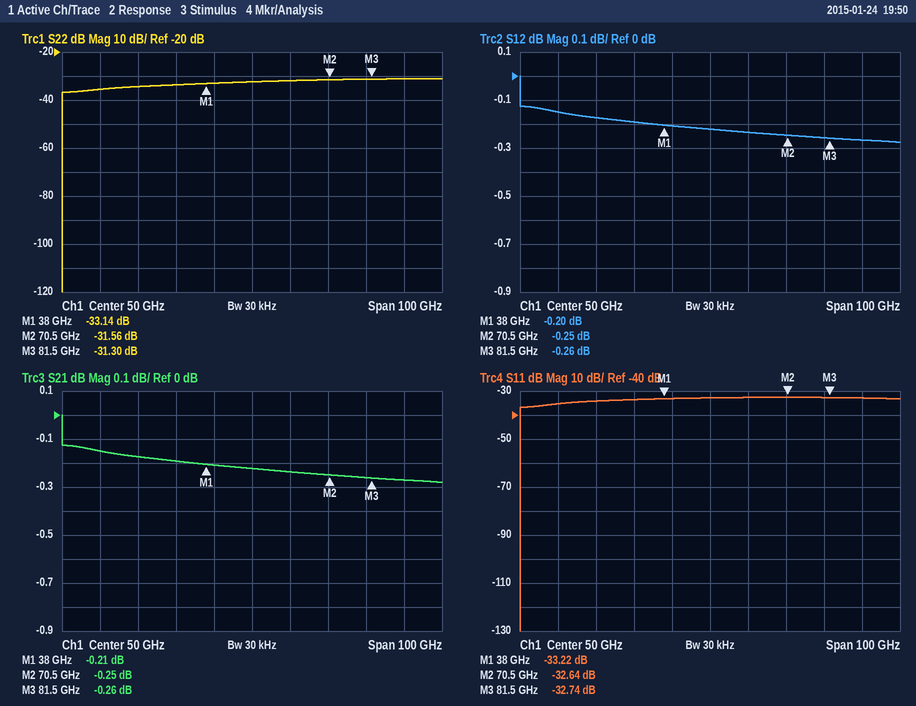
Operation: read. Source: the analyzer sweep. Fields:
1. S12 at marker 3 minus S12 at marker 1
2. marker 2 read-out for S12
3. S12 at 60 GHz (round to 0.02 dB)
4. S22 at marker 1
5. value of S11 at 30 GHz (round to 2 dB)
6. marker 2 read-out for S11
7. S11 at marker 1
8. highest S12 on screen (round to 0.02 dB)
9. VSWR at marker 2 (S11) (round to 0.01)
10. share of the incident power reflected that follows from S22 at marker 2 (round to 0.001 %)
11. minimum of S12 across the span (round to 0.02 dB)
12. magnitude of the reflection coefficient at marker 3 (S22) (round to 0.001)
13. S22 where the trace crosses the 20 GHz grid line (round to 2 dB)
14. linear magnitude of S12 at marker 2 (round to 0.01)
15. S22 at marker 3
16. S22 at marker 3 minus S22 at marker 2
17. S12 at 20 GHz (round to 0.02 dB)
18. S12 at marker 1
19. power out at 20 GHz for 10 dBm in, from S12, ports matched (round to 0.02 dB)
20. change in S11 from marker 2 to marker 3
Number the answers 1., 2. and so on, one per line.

1. -0.06 dB
2. -0.25 dB
3. -0.24 dB
4. -33.14 dB
5. -34 dB
6. -32.64 dB
7. -33.22 dB
8. 0.00 dB
9. 1.05
10. 0.070 %
11. -0.28 dB
12. 0.027
13. -34 dB
14. 0.97
15. -31.30 dB
16. 0.26 dB
17. -0.18 dB
18. -0.20 dB
19. 9.82 dBm
20. -0.10 dB
